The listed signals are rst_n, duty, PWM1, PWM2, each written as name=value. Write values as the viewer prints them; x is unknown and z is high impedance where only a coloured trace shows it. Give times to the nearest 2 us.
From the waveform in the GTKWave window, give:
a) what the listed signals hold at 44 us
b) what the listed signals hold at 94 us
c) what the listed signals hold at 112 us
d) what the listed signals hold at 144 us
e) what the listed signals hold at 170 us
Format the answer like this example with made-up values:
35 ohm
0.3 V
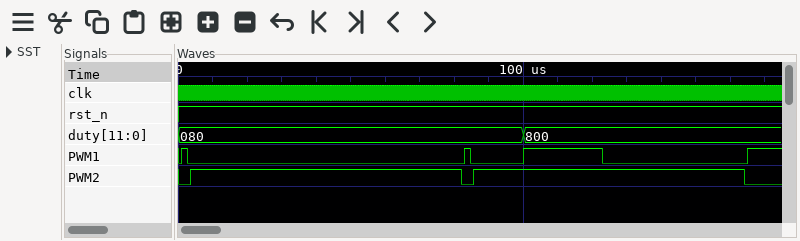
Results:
rst_n=1, duty=080, PWM1=0, PWM2=1
rst_n=1, duty=080, PWM1=0, PWM2=1
rst_n=1, duty=800, PWM1=1, PWM2=1
rst_n=1, duty=800, PWM1=0, PWM2=1
rst_n=1, duty=800, PWM1=1, PWM2=0
